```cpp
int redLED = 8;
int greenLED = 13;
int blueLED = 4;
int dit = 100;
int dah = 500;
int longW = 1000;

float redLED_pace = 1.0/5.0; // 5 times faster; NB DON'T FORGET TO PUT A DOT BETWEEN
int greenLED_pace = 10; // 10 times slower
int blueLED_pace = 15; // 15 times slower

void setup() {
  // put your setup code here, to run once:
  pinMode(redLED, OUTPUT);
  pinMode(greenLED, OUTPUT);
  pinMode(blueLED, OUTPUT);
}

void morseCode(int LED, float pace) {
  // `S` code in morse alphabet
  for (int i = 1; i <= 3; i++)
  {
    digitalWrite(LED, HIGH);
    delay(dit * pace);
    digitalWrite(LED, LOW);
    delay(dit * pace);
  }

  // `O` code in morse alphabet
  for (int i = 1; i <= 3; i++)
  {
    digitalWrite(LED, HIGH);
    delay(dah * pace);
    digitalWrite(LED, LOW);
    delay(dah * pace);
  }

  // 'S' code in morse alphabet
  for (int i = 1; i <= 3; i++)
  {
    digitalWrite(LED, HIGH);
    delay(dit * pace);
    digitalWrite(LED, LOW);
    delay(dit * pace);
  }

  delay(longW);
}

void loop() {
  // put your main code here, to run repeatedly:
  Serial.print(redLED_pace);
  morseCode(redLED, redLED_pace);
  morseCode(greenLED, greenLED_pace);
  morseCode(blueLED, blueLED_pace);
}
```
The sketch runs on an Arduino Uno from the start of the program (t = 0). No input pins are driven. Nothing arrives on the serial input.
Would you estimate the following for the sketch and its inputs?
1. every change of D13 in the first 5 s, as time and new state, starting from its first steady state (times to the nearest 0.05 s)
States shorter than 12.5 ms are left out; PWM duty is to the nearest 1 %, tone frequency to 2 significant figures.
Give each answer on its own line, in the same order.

0 s low; 1.85 s high; 2.85 s low; 3.85 s high; 4.85 s low
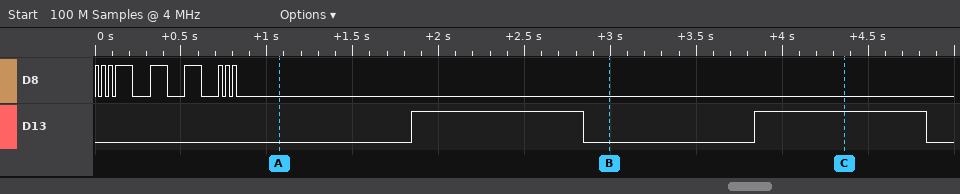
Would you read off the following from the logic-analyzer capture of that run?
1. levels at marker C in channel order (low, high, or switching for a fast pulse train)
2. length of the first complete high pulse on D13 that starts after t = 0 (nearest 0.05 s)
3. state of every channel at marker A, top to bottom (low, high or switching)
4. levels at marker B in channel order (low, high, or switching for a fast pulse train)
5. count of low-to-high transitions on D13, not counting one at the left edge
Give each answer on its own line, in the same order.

D8 low, D13 high
1.00 s
D8 low, D13 low
D8 low, D13 low
2
